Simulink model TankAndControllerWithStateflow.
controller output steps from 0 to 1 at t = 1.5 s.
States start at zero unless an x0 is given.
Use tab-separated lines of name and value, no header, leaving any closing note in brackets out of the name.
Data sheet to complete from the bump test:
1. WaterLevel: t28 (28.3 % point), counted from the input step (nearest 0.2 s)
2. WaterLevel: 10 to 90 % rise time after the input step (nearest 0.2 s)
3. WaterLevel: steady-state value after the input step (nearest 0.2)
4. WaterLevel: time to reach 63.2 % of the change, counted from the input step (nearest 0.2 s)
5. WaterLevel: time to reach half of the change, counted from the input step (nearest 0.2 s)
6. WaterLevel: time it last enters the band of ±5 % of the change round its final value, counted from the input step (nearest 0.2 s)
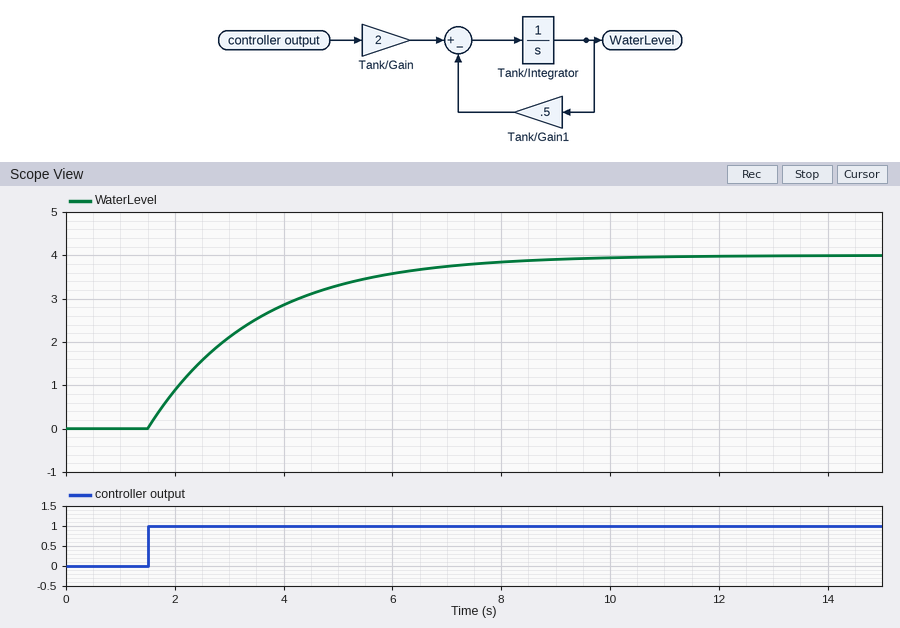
WaterLevel: t28 (28.3 % point), counted from the input step	0.6 s
WaterLevel: 10 to 90 % rise time after the input step	4.4 s
WaterLevel: steady-state value after the input step	4.0
WaterLevel: time to reach 63.2 % of the change, counted from the input step	2.0 s
WaterLevel: time to reach half of the change, counted from the input step	1.4 s
WaterLevel: time it last enters the band of ±5 % of the change round its final value, counted from the input step	6.0 s
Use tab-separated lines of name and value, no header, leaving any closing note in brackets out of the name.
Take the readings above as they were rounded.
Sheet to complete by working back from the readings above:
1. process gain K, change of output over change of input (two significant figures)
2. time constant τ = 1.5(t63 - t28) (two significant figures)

process gain K, change of output over change of input	4.0
time constant τ = 1.5(t63 - t28)	2.1 s
